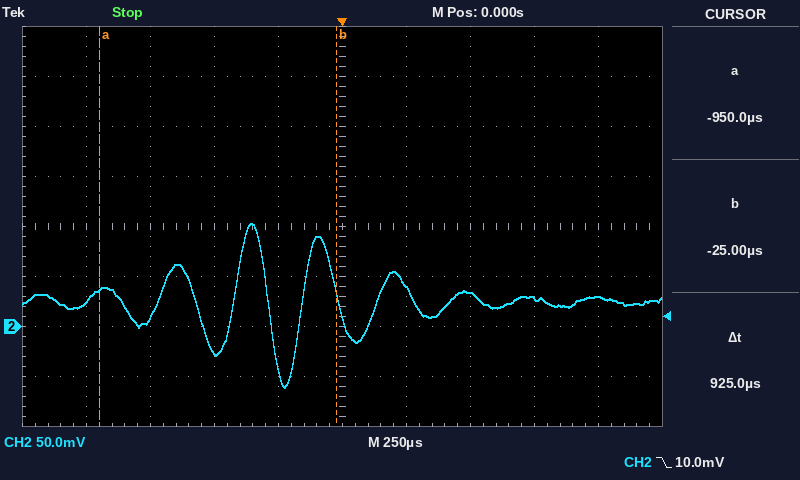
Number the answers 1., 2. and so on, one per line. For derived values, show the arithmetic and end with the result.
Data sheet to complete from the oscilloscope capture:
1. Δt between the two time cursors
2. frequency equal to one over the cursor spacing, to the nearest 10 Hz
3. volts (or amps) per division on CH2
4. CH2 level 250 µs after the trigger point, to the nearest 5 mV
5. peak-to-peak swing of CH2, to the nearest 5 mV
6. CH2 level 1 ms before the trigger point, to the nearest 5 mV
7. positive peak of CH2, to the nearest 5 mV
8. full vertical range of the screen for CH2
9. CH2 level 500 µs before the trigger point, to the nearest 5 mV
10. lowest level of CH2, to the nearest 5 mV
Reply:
1. 925 µs
2. 1 / 925 µs ≈ 1.08 kHz
3. 50 mV
4. 40 mV
5. 105 mV − (-60 mV) = 165 mV
6. 25 mV
7. 105 mV
8. 400 mV
9. -25 mV
10. -60 mV
